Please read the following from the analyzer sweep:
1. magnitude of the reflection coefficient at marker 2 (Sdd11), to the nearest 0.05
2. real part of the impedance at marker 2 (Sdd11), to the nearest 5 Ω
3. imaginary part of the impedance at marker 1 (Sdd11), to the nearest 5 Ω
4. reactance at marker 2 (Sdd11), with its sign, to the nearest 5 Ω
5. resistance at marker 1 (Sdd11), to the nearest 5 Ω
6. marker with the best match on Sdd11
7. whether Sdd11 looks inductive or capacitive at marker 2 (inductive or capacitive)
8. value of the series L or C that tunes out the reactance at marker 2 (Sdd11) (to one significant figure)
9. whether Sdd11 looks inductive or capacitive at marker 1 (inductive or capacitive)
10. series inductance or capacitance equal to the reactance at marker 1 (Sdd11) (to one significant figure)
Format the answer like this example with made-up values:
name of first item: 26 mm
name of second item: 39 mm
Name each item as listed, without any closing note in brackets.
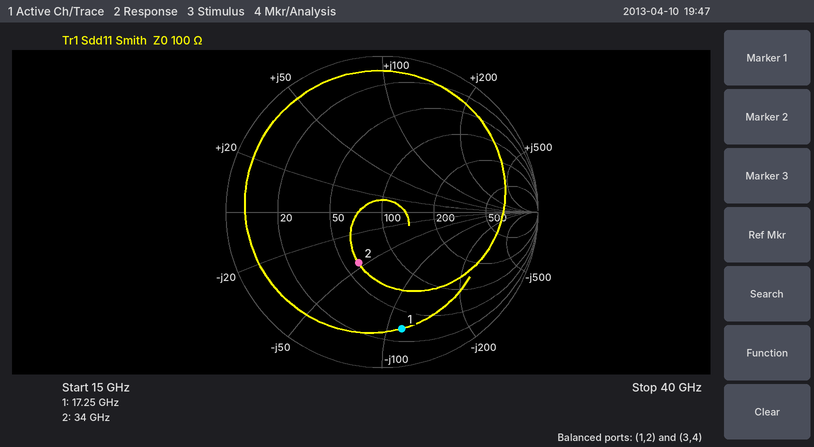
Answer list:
magnitude of the reflection coefficient at marker 2 (Sdd11), to the nearest 0.05: 0.35
real part of the impedance at marker 2 (Sdd11), to the nearest 5 Ω: 60 Ω
imaginary part of the impedance at marker 1 (Sdd11), to the nearest 5 Ω: -115 Ω
reactance at marker 2 (Sdd11), with its sign, to the nearest 5 Ω: -45 Ω
resistance at marker 1 (Sdd11), to the nearest 5 Ω: 30 Ω
marker with the best match on Sdd11: marker 2
whether Sdd11 looks inductive or capacitive at marker 2: capacitive
value of the series L or C that tunes out the reactance at marker 2 (Sdd11): 200 pH
whether Sdd11 looks inductive or capacitive at marker 1: capacitive
series inductance or capacitance equal to the reactance at marker 1 (Sdd11): 80 fF
